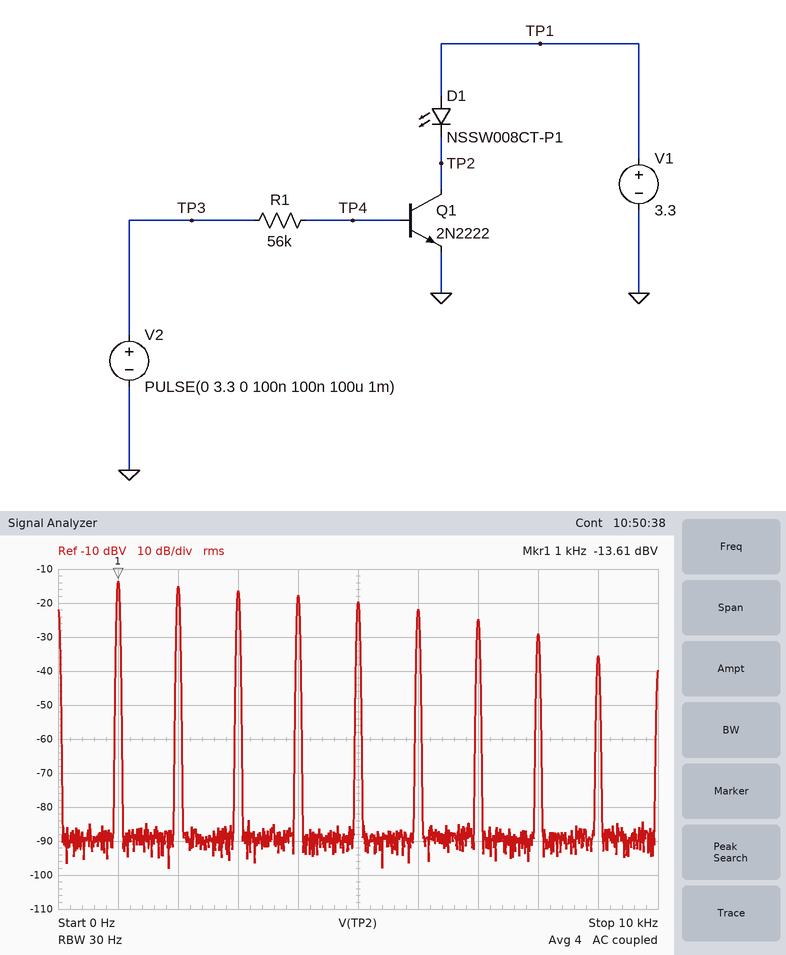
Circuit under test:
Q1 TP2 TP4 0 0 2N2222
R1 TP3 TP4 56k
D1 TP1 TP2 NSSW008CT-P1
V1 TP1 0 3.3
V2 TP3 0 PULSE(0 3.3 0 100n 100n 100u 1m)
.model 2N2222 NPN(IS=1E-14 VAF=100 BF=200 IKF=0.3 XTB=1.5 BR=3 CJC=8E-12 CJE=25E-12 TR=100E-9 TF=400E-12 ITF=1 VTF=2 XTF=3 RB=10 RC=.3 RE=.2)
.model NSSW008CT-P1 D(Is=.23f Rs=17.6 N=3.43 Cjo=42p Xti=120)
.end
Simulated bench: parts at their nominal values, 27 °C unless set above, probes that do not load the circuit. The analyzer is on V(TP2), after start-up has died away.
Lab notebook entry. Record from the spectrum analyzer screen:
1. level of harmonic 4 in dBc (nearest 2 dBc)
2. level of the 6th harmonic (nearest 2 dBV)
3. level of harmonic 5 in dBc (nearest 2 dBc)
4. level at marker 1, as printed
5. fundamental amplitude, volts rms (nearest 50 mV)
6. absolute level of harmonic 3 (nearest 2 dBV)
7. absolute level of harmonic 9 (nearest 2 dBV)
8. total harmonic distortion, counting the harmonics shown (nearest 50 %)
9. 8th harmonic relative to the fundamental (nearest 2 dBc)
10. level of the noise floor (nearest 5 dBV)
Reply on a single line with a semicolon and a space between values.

-4 dBc; -22 dBV; -6 dBc; -13.61 dBV; 200 mV; -16 dBV; -36 dBV; 150 %; -16 dBc; -90 dBV
